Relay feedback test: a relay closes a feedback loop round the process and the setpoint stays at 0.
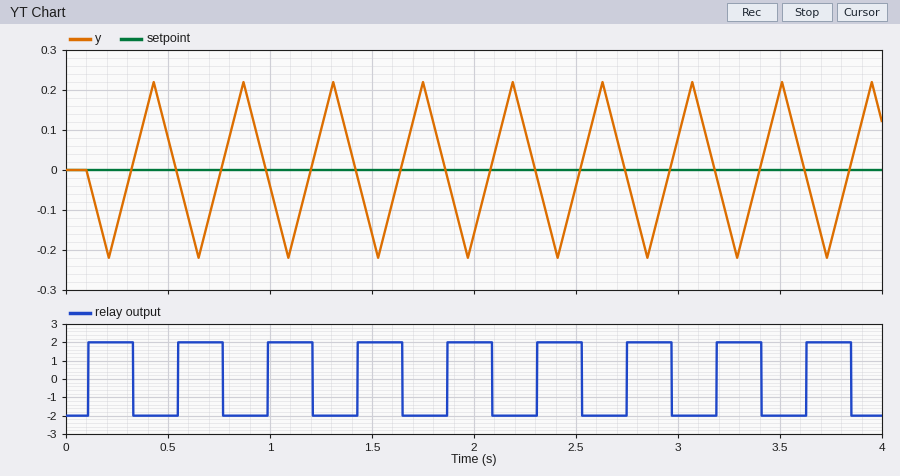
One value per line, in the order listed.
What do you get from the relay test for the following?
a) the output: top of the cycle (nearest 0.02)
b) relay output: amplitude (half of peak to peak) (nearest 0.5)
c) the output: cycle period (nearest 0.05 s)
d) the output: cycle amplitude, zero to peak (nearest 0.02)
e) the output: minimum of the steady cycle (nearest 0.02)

0.22
2.0
0.45 s
0.22
-0.22
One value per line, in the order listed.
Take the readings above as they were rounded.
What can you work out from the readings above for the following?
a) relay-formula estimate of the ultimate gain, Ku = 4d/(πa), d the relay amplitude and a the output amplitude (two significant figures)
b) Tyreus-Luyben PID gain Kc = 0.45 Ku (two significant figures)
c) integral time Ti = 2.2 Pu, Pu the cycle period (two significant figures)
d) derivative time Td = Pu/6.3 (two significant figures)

12
5.4
0.99 s
0.071 s
